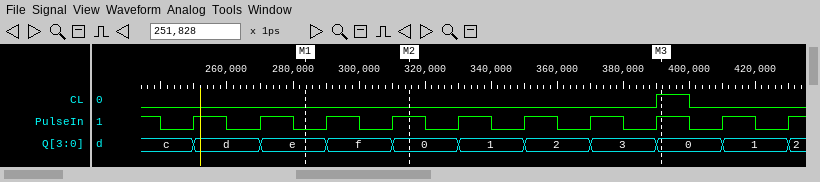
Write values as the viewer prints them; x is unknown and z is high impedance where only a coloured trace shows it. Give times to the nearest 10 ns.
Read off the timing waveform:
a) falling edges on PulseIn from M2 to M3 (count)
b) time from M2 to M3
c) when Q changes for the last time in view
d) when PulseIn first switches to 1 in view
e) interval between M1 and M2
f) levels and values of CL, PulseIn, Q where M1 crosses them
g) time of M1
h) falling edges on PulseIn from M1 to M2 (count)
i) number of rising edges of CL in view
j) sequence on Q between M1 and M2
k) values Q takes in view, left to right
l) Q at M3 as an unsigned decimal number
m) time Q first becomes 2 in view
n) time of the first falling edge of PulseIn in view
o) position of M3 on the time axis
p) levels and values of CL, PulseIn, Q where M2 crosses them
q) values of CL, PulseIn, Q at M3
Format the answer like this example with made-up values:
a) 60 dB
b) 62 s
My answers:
a) 4
b) 80 ns
c) 430 ns
d) 250 ns
e) 30 ns
f) CL=0, PulseIn=0, Q=e
g) 280 ns
h) 1
i) 1
j) e, f, 0
k) c, d, e, f, 0, 1, 2, 3, 0, 1, 2
l) 0
m) 350 ns
n) 240 ns
o) 390 ns
p) CL=0, PulseIn=1, Q=0
q) CL=1, PulseIn=1, Q=0
